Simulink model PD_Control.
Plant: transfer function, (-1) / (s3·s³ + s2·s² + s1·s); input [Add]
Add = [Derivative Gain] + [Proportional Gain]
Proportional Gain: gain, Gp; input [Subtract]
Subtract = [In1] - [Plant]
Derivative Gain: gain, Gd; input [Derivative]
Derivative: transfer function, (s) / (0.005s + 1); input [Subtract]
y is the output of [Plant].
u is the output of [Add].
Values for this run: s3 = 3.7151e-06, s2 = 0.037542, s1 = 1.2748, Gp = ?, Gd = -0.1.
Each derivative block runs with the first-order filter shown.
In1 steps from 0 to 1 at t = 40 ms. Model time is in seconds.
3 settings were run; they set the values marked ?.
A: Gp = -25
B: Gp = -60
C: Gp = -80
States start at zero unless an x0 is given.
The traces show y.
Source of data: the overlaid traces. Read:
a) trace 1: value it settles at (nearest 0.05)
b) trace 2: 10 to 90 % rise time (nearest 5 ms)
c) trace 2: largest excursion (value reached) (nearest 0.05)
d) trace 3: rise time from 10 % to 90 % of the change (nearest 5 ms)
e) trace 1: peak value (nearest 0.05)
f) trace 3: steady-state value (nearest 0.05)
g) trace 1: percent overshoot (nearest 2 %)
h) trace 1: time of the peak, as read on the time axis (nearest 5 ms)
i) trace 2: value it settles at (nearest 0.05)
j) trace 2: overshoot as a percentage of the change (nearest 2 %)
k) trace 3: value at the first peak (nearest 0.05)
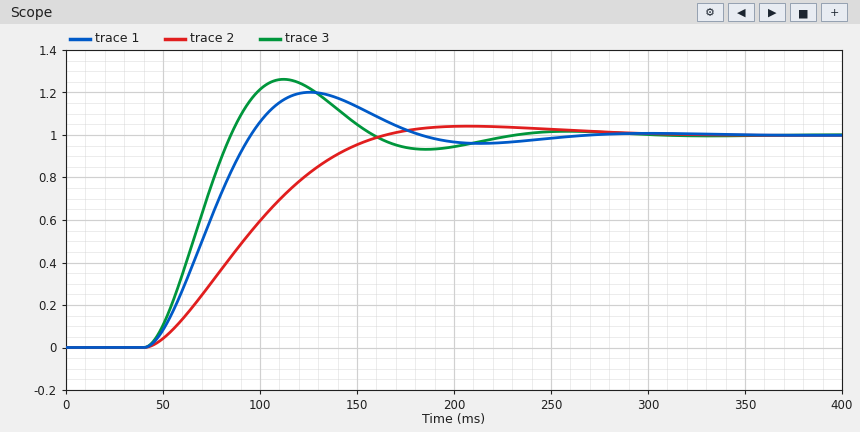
1.00
80 ms
1.05
30 ms
1.20
1.00
20 %
125 ms
1.00
4 %
1.25
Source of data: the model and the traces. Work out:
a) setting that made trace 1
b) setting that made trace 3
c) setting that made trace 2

B
C
A
